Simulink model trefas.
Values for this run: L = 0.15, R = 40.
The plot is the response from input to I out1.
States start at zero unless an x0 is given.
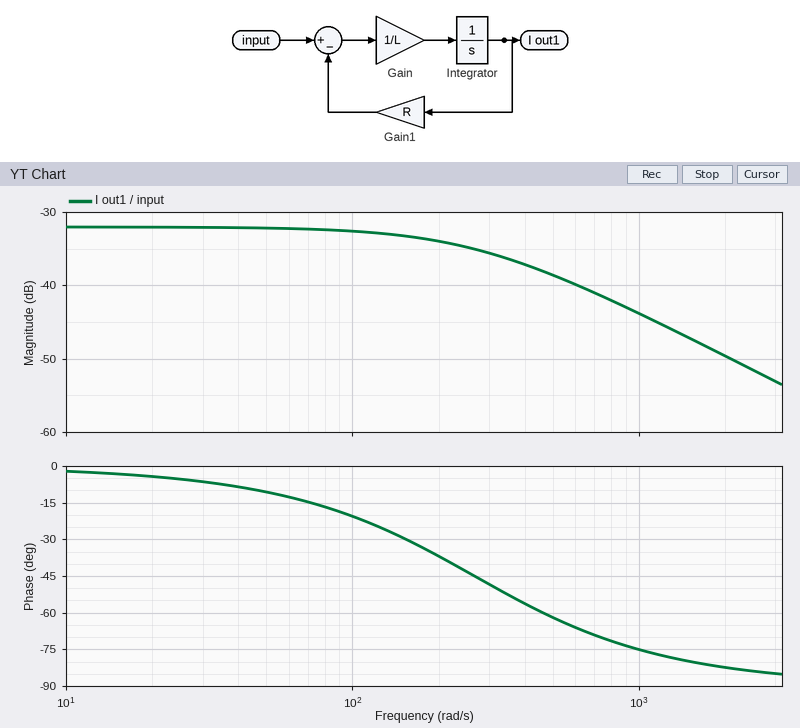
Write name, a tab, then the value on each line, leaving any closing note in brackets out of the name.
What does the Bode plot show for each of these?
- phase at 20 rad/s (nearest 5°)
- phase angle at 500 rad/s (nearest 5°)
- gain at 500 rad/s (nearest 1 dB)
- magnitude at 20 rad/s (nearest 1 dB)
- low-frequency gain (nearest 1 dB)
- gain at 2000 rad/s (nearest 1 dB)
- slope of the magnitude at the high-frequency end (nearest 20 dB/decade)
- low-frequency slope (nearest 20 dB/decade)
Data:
phase at 20 rad/s	-5°
phase angle at 500 rad/s	-60°
gain at 500 rad/s	-39 dB
magnitude at 20 rad/s	-32 dB
low-frequency gain	-32 dB
gain at 2000 rad/s	-50 dB
slope of the magnitude at the high-frequency end	-20 dB/decade
low-frequency slope	0 dB/decade
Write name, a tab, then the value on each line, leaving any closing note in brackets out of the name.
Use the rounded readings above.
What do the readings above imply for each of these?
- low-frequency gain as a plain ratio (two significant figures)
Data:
low-frequency gain as a plain ratio	0.025
